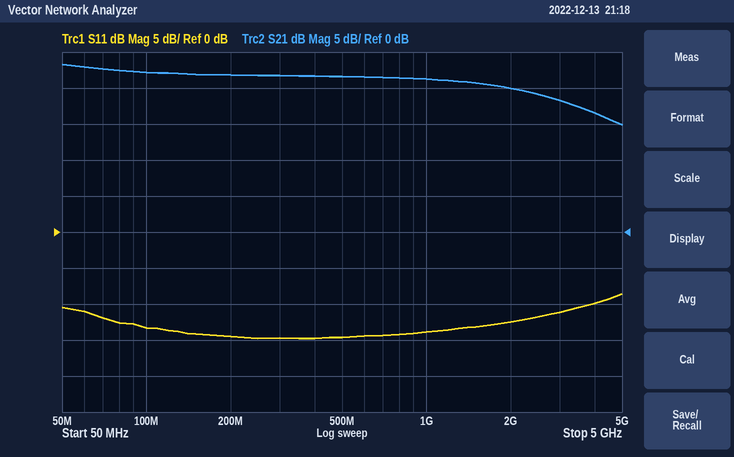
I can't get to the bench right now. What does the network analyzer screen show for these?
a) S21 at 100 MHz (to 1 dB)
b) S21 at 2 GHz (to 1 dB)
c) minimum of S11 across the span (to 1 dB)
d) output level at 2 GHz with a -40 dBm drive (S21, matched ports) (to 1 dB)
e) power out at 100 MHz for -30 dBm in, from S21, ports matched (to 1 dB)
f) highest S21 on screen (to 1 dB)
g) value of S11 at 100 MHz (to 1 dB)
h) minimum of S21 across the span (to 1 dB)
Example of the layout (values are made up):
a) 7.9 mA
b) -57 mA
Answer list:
a) 22 dB
b) 20 dB
c) -15 dB
d) -20 dBm
e) -8 dBm
f) 23 dB
g) -13 dB
h) 15 dB
